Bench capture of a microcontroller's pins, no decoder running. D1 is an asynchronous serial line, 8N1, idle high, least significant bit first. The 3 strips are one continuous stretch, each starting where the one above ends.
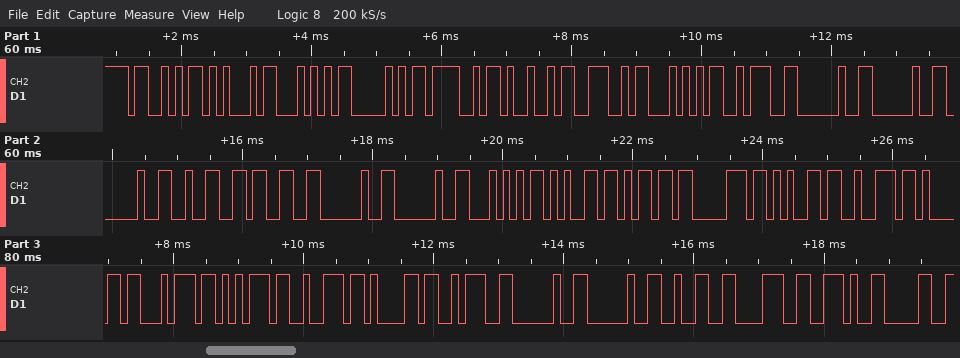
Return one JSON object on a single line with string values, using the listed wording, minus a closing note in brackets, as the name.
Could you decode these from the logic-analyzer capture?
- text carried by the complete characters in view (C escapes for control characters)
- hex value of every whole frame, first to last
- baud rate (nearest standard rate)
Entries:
{"text carried by the complete characters in view": "\"SETPOINT:   23  Temperatura:  28.0\"", "hex value of every whole frame, first to last": "53 45 54 50 4F 49 4E 54 3A 20 20 20 32 33 20 20 54 65 6D 70 65 72 61 74 75 72 61 3A 20 20 32 38 2E 30", "baud rate": "9600 baud"}
